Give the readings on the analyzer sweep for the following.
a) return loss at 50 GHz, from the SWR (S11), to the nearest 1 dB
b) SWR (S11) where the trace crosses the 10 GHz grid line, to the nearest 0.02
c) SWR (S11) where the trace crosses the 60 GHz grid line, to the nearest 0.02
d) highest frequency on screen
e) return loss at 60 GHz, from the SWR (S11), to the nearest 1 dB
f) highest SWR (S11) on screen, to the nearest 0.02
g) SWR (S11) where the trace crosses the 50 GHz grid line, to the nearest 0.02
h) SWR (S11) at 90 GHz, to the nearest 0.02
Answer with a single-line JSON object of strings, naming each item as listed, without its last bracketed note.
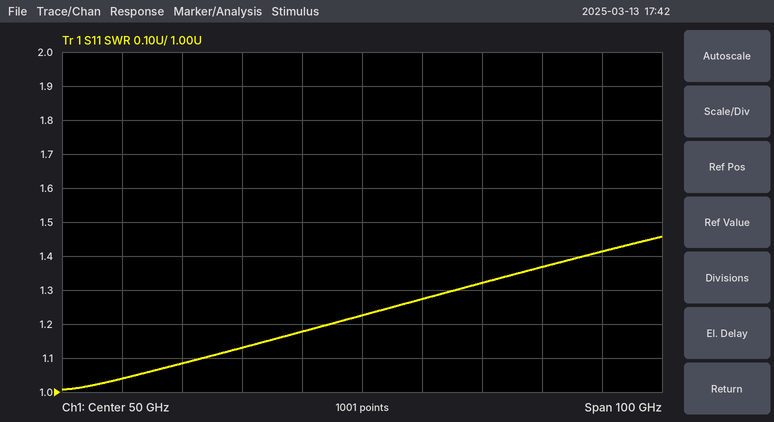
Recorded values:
{"return loss at 50 GHz, from the SWR (S11), to the nearest 1 dB": "20 dB", "SWR (S11) where the trace crosses the 10 GHz grid line, to the nearest 0.02": "1.04", "SWR (S11) where the trace crosses the 60 GHz grid line, to the nearest 0.02": "1.28", "highest frequency on screen": "100 GHz", "return loss at 60 GHz, from the SWR (S11), to the nearest 1 dB": "18 dB", "highest SWR (S11) on screen, to the nearest 0.02": "1.46", "SWR (S11) where the trace crosses the 50 GHz grid line, to the nearest 0.02": "1.22", "SWR (S11) at 90 GHz, to the nearest 0.02": "1.42"}
